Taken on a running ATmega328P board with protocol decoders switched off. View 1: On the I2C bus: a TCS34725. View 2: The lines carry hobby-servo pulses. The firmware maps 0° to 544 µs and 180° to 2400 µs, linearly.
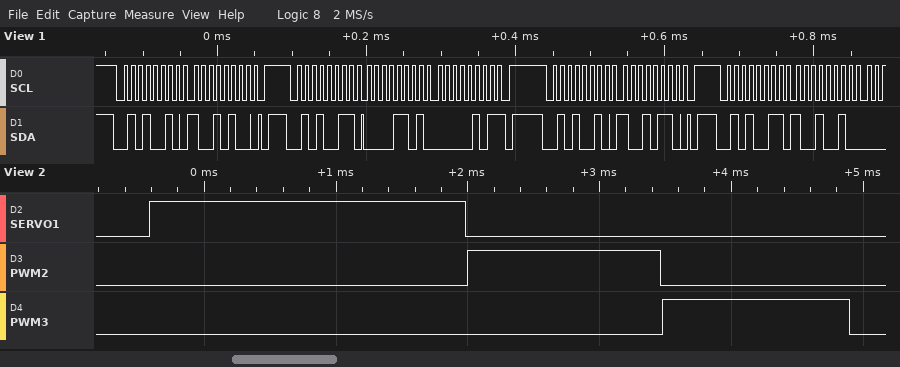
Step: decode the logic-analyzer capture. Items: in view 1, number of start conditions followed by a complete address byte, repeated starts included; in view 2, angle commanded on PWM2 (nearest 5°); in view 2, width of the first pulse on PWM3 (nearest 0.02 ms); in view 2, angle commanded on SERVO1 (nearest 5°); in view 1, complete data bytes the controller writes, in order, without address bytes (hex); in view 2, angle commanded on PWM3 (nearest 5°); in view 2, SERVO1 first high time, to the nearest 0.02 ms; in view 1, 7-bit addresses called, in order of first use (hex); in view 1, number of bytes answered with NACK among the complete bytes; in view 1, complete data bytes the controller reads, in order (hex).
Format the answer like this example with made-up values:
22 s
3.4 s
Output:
4
90°
1.42 ms
180°
94 96
85°
2.40 ms
0x29
1
0D 05 92
